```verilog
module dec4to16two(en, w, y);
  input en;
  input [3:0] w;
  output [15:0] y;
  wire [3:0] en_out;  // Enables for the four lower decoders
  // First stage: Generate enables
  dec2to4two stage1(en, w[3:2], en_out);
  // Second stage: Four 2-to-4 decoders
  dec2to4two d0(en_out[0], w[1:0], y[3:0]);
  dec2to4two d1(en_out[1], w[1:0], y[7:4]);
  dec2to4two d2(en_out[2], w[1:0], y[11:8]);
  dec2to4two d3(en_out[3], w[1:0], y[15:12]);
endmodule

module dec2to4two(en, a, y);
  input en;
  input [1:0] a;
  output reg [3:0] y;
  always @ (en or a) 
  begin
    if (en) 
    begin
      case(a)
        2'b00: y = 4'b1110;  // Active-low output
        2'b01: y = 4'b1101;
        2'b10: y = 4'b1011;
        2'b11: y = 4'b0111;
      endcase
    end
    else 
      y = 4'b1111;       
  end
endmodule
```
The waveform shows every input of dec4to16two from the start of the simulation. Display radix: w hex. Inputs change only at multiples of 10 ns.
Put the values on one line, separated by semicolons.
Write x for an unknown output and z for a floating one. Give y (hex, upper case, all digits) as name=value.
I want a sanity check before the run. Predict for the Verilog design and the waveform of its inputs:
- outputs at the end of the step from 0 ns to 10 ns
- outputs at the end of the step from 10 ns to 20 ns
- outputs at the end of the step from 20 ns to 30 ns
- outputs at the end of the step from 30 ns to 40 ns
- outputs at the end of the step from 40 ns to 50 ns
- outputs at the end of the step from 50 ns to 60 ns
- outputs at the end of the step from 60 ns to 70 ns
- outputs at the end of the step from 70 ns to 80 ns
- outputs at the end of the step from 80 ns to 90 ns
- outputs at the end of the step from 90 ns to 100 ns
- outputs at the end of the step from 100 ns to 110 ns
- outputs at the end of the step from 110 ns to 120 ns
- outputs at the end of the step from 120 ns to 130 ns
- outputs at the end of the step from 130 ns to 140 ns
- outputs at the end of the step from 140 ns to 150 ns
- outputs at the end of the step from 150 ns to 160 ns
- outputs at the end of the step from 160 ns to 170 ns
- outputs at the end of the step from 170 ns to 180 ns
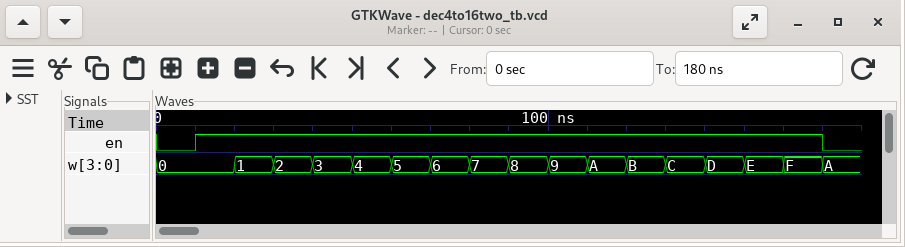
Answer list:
y=EEEE; y=EEEF; y=DDDF; y=BBBF; y=777F; y=EEFE; y=DDFD; y=BBFB; y=77F7; y=EFEE; y=DFDD; y=BFBB; y=7F77; y=FEEE; y=FDDD; y=FBBB; y=F777; y=BBBB
